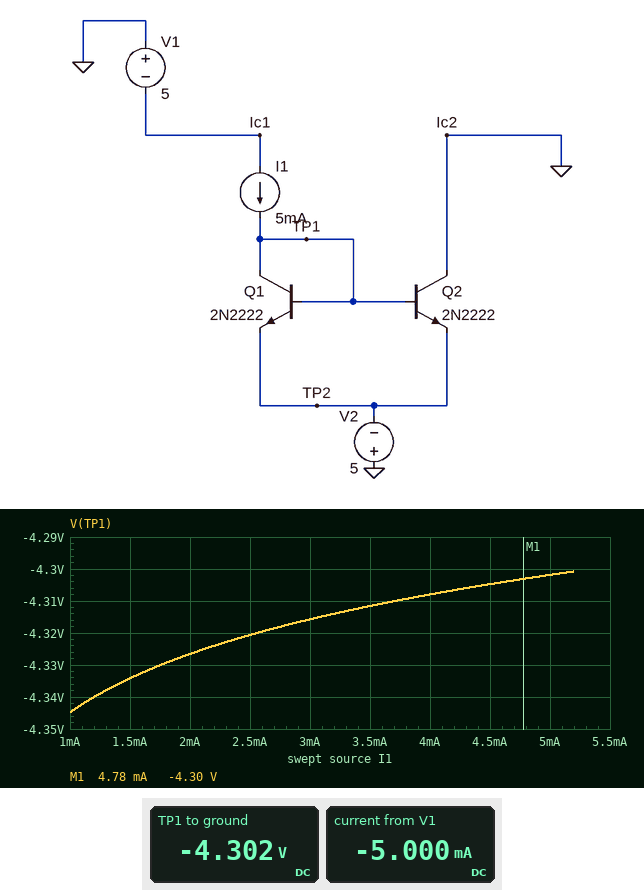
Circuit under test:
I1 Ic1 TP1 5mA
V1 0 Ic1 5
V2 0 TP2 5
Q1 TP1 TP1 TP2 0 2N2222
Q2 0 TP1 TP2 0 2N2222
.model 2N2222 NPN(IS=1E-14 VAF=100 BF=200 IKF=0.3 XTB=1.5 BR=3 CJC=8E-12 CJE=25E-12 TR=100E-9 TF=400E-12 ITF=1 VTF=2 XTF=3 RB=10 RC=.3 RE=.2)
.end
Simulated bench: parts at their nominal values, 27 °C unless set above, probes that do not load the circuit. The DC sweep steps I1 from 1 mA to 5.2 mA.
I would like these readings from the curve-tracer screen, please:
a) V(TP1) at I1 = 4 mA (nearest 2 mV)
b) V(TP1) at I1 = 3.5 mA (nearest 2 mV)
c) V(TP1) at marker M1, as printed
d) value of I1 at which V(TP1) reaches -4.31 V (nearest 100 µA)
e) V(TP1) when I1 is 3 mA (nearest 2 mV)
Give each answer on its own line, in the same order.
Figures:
-4.308 V
-4.312 V
-4.30 V
3.7 mA
-4.316 V
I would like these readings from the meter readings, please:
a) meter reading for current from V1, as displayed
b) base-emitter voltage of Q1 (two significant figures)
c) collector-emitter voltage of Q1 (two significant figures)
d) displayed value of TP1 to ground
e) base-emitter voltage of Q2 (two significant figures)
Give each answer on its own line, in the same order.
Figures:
-5.000 mA
700 mV
700 mV
-4.302 V
700 mV
